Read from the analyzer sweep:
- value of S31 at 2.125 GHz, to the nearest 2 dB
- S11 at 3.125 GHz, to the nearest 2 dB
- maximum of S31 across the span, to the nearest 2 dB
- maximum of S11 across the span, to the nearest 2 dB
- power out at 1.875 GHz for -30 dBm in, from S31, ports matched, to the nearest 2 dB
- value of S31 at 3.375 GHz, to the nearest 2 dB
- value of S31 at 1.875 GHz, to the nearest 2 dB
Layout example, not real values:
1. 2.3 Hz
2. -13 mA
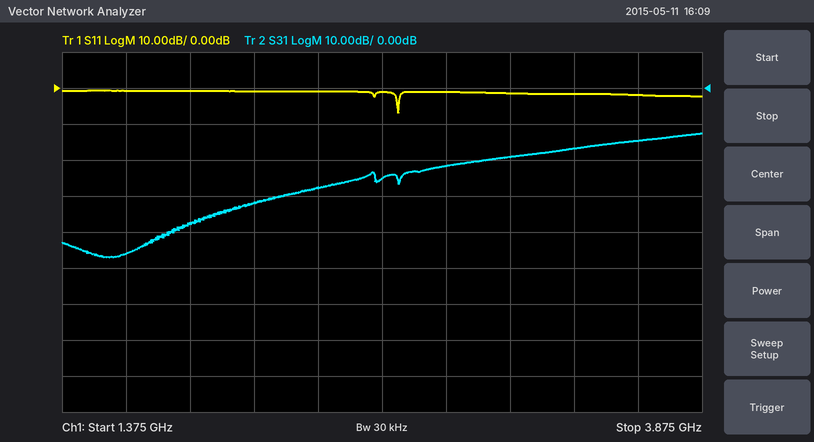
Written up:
1. -32 dB
2. -2 dB
3. -12 dB
4. 0 dB
5. -68 dBm
6. -16 dB
7. -38 dB
